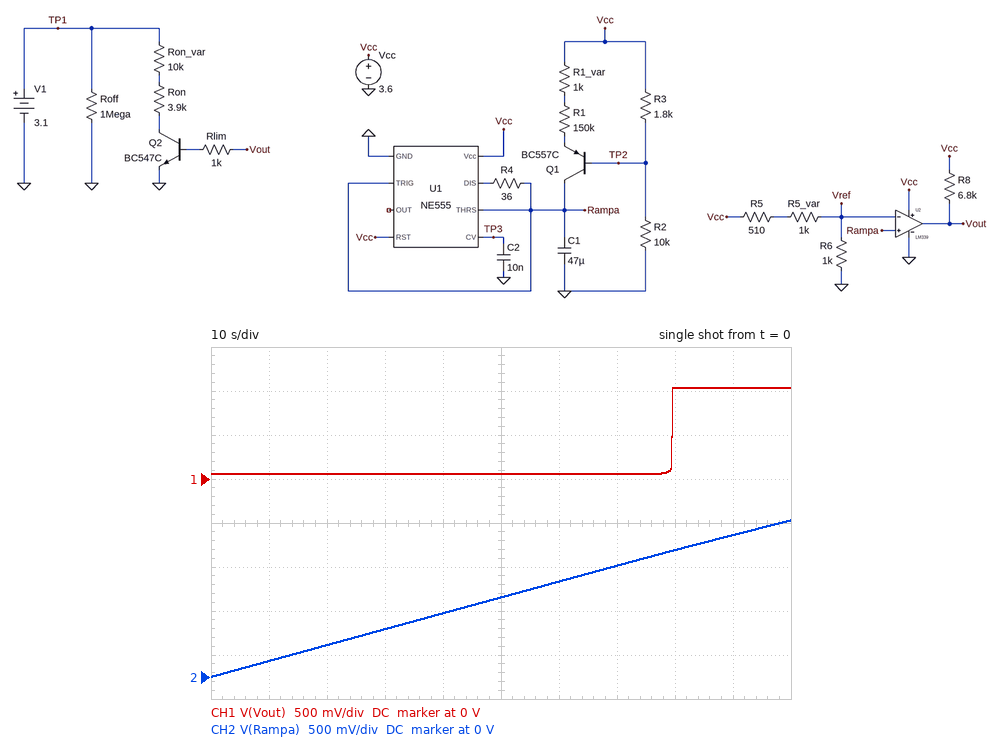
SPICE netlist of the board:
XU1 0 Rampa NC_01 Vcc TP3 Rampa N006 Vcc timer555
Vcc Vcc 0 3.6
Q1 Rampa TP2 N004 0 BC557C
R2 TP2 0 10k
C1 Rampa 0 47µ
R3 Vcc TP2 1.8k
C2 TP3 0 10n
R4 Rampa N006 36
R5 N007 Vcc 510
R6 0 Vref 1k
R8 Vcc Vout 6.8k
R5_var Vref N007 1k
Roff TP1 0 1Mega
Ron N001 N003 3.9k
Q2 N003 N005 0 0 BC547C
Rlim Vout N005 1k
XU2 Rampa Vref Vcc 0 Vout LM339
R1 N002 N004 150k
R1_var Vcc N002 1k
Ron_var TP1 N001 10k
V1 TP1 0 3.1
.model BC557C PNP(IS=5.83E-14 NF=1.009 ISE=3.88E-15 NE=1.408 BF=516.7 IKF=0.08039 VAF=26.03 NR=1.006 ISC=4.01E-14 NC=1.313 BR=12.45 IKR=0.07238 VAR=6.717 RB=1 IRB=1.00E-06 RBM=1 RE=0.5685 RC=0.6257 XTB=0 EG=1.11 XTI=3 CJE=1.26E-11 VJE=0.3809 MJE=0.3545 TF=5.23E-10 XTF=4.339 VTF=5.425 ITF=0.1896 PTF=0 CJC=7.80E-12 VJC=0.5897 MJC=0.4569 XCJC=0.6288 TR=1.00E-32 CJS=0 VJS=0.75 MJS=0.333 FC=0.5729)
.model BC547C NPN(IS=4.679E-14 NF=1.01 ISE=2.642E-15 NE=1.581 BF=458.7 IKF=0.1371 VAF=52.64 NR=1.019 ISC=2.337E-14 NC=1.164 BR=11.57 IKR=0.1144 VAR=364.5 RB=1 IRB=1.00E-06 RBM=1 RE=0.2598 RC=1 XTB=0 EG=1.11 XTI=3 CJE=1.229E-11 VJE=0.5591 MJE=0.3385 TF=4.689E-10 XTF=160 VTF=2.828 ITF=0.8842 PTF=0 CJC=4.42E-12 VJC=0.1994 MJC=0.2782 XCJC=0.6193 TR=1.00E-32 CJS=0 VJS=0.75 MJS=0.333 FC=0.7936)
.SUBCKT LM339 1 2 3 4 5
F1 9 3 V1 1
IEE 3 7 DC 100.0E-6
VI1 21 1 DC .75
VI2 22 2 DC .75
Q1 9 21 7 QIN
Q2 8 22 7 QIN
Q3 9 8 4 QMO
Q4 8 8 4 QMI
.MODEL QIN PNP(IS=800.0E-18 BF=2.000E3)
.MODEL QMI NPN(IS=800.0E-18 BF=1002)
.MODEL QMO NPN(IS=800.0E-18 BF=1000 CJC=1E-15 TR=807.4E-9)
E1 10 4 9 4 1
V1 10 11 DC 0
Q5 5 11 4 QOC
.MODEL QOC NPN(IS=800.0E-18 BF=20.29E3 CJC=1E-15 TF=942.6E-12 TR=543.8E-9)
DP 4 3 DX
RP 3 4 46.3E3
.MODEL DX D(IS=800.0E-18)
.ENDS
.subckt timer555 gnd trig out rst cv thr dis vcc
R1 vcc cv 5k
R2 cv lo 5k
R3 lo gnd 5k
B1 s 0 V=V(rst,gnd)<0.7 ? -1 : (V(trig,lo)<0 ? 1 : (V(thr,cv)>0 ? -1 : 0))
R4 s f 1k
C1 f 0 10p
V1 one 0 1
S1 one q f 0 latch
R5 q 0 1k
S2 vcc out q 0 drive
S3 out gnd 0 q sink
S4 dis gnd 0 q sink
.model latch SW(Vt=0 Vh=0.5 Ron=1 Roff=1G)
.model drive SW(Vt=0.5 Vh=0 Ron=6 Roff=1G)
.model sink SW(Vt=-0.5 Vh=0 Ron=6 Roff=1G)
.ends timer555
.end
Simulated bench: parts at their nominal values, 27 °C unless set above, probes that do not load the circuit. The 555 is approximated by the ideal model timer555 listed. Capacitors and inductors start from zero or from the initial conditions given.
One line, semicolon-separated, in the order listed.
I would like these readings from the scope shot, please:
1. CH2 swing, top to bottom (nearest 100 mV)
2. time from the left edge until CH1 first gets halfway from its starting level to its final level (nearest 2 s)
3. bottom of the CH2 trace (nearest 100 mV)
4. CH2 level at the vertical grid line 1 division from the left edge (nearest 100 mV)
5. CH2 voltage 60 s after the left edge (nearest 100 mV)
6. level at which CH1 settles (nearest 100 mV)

1.8 V; 80 s; 0 V; 200 mV; 1.1 V; 1.0 V
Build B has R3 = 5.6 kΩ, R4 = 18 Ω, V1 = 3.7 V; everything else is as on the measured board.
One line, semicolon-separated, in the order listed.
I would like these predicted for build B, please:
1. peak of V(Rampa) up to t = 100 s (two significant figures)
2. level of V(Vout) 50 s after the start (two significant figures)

2.4 V; 1.0 V
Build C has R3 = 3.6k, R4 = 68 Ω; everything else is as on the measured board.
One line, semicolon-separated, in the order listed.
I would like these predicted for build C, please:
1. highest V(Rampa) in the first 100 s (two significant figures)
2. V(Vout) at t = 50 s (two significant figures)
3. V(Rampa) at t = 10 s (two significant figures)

2.4 V; 1.0 V; 700 mV
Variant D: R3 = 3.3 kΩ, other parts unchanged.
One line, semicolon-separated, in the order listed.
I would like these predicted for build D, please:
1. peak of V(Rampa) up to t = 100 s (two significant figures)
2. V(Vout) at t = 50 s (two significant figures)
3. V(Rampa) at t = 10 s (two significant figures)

2.4 V; 1.0 V; 620 mV
